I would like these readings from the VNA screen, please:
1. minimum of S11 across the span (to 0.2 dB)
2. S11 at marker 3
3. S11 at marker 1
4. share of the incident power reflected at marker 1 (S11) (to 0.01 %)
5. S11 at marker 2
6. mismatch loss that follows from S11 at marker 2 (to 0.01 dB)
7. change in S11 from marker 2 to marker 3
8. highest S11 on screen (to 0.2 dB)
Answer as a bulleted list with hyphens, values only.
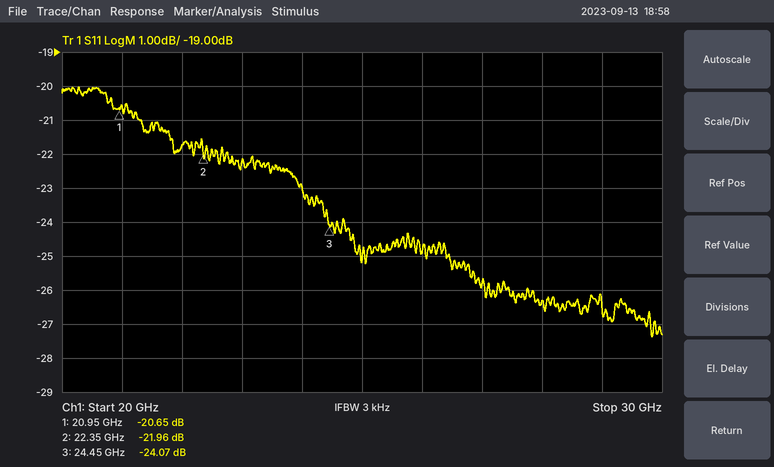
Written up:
- -27.4 dB
- -24.07 dB
- -20.65 dB
- 0.86 %
- -21.96 dB
- 0.03 dB
- -2.11 dB
- -20.0 dB
